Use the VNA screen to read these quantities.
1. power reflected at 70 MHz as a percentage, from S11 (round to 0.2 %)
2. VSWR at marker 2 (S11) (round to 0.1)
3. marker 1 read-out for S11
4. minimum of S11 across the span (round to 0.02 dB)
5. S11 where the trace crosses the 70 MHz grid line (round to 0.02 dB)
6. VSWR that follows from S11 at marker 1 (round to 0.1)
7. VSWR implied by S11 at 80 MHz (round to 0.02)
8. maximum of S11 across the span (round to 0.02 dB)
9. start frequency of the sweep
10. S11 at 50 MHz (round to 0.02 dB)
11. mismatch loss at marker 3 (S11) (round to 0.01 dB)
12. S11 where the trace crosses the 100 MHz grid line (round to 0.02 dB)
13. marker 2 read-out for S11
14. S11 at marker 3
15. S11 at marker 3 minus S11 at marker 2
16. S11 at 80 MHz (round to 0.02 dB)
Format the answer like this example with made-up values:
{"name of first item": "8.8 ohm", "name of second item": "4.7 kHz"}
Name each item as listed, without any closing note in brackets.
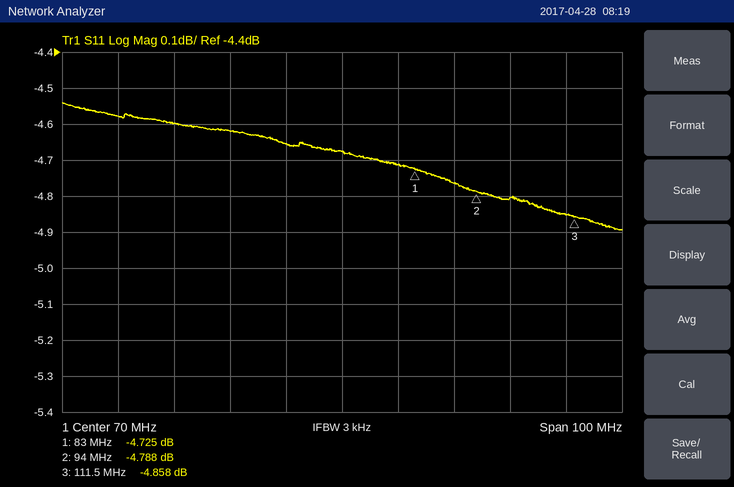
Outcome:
{"power reflected at 70 MHz as a percentage, from S11": "34.0 %", "VSWR at marker 2 (S11)": "3.7", "marker 1 read-out for S11": "-4.725 dB", "minimum of S11 across the span": "-4.90 dB", "S11 where the trace crosses the 70 MHz grid line": "-4.68 dB", "VSWR that follows from S11 at marker 1": "3.8", "VSWR implied by S11 at 80 MHz": "3.78", "maximum of S11 across the span": "-4.54 dB", "start frequency of the sweep": "20 MHz", "S11 at 50 MHz": "-4.62 dB", "mismatch loss at marker 3 (S11)": "1.72 dB", "S11 where the trace crosses the 100 MHz grid line": "-4.80 dB", "marker 2 read-out for S11": "-4.788 dB", "S11 at marker 3": "-4.858 dB", "S11 at marker 3 minus S11 at marker 2": "-0.070 dB", "S11 at 80 MHz": "-4.72 dB"}
